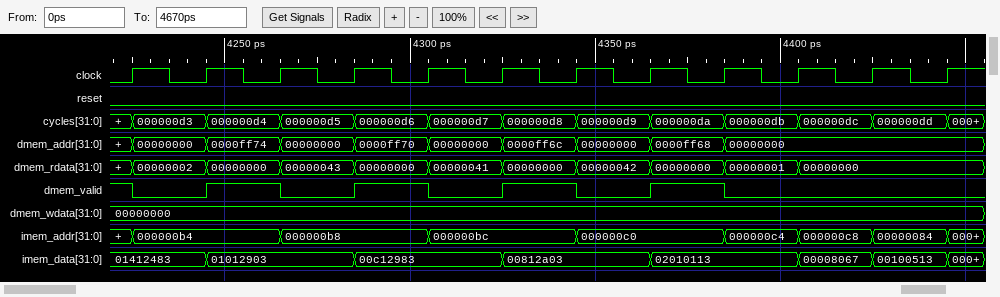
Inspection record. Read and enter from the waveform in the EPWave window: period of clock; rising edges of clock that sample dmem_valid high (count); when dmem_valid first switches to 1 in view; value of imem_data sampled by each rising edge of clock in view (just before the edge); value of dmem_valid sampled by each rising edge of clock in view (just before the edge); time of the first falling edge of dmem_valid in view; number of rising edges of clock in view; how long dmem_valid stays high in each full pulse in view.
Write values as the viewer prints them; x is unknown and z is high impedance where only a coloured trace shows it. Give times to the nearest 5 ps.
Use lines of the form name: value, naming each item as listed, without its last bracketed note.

period of clock: 20 ps
rising edges of clock that sample dmem_valid high: 5
when dmem_valid first switches to 1 in view: 4245 ps
value of imem_data sampled by each rising edge of clock in view: 01412483, 01412483, 01012903, 01012903, 00c12983, 00c12983, 00812a03, 00812a03, 02010113, 02010113, 00008067, 00100513
value of dmem_valid sampled by each rising edge of clock in view: 1 0 1 0 1 0 1 0 1 0 0 0
time of the first falling edge of dmem_valid in view: 4225 ps
number of rising edges of clock in view: 12
how long dmem_valid stays high in each full pulse in view: 20 ps, 20 ps, 20 ps, 20 ps
